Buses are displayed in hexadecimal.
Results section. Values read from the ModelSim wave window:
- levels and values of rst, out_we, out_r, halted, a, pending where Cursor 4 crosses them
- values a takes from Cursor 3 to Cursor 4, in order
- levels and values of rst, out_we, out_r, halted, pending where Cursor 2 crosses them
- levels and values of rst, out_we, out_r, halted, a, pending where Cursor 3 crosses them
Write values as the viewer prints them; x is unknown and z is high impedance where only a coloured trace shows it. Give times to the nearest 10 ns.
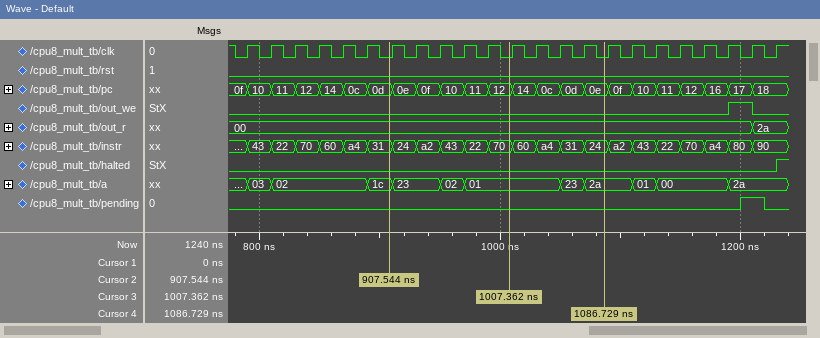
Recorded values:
rst=0, out_we=0, out_r=00, halted=0, a=2a, pending=0
01, 23, 2a
rst=0, out_we=0, out_r=00, halted=0, pending=0
rst=0, out_we=0, out_r=00, halted=0, a=01, pending=0
